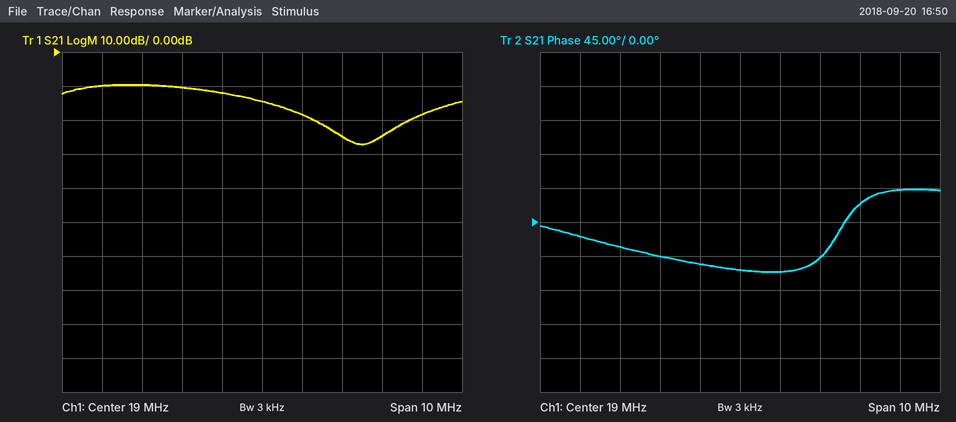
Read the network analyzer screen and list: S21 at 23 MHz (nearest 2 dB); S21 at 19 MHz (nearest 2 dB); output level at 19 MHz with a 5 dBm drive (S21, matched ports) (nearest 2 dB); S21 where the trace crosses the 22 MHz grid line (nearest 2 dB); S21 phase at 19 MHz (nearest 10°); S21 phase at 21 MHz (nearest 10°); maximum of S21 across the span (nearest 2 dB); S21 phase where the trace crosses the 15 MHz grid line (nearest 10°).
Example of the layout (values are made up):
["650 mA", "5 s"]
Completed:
["-18 dB", "-14 dB", "-10 dBm", "-24 dB", "-60°", "-50°", "-10 dB", "-20°"]
